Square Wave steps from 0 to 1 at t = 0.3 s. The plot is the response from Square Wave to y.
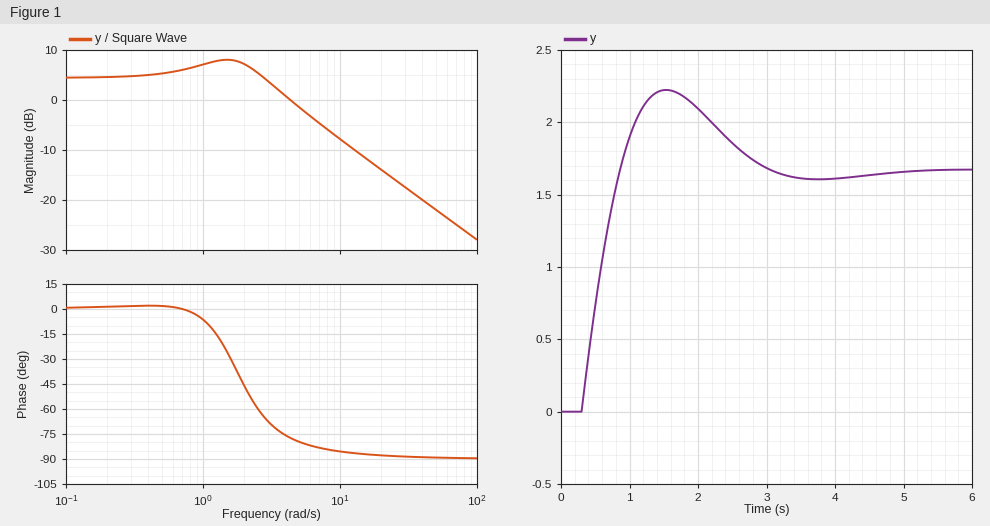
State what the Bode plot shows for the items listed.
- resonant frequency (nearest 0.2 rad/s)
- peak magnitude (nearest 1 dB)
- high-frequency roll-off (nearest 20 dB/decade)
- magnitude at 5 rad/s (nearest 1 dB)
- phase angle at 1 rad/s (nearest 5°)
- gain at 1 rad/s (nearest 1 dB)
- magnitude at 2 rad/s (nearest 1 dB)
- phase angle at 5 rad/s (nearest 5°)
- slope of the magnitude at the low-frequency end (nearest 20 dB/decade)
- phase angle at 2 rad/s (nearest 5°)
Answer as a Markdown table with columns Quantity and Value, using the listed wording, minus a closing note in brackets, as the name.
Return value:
| Quantity | Value |
|---|---|
| resonant frequency | 1.4 rad/s |
| peak magnitude | 8 dB |
| high-frequency roll-off | -20 dB/decade |
| magnitude at 5 rad/s | -1 dB |
| phase angle at 1 rad/s | -5° |
| gain at 1 rad/s | 7 dB |
| magnitude at 2 rad/s | 7 dB |
| phase angle at 5 rad/s | -80° |
| slope of the magnitude at the low-frequency end | 0 dB/decade |
| phase angle at 2 rad/s | -45° |
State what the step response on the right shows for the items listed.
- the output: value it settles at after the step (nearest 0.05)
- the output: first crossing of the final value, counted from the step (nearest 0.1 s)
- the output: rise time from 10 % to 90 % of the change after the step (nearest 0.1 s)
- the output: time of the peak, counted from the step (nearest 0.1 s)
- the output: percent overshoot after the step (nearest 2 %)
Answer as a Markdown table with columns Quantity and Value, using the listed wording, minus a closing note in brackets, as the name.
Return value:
| Quantity | Value |
|---|---|
| the output: value it settles at after the step | 1.65 |
| the output: first crossing of the final value, counted from the step | 0.6 s |
| the output: rise time from 10 % to 90 % of the change after the step | 0.4 s |
| the output: time of the peak, counted from the step | 1.2 s |
| the output: percent overshoot after the step | 34 % |
